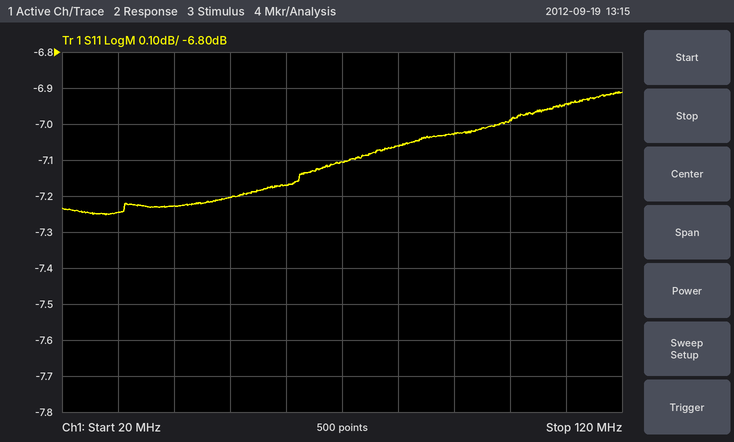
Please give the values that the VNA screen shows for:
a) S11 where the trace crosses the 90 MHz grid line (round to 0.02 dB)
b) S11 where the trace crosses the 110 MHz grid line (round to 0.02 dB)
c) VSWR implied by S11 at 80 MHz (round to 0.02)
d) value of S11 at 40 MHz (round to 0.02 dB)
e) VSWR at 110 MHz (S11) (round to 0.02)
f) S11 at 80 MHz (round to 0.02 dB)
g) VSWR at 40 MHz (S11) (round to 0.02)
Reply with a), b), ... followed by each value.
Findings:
a) -7.02 dB
b) -6.94 dB
c) 2.60
d) -7.22 dB
e) 2.64
f) -7.06 dB
g) 2.54
